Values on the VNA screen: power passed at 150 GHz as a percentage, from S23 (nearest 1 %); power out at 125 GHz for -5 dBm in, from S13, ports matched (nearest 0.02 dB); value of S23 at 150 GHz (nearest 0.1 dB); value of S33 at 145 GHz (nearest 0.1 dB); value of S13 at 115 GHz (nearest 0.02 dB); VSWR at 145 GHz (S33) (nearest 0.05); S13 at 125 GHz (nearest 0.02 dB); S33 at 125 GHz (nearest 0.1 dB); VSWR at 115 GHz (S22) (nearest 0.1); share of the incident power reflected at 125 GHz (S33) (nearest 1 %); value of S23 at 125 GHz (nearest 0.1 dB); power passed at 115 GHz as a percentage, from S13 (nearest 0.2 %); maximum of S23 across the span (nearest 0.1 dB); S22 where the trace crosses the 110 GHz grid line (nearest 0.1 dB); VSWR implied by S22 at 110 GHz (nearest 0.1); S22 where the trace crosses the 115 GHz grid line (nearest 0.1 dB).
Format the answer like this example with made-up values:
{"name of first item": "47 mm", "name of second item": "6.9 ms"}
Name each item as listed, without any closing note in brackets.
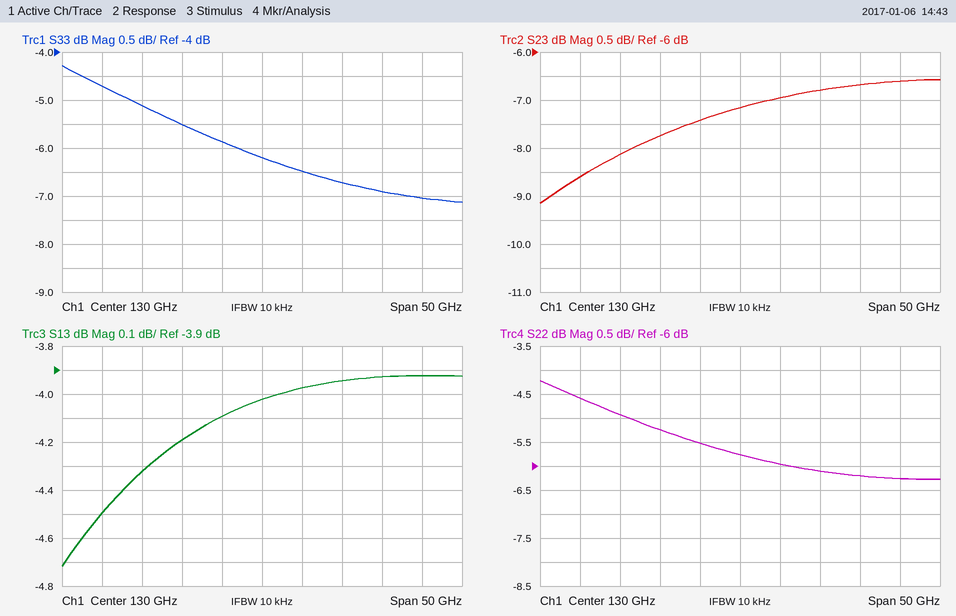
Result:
{"power passed at 150 GHz as a percentage, from S23": "22 %", "power out at 125 GHz for -5 dBm in, from S13, ports matched": "-9.10 dBm", "value of S23 at 150 GHz": "-6.6 dB", "value of S33 at 145 GHz": "-6.9 dB", "value of S13 at 115 GHz": "-4.32 dB", "VSWR at 145 GHz (S33)": "2.65", "S13 at 125 GHz": "-4.10 dB", "S33 at 125 GHz": "-5.9 dB", "VSWR at 115 GHz (S22)": "3.6", "share of the incident power reflected at 125 GHz (S33)": "26 %", "value of S23 at 125 GHz": "-7.4 dB", "power passed at 115 GHz as a percentage, from S13": "37.0 %", "maximum of S23 across the span": "-6.6 dB", "S22 where the trace crosses the 110 GHz grid line": "-4.6 dB", "VSWR implied by S22 at 110 GHz": "3.9", "S22 where the trace crosses the 115 GHz grid line": "-4.9 dB"}
